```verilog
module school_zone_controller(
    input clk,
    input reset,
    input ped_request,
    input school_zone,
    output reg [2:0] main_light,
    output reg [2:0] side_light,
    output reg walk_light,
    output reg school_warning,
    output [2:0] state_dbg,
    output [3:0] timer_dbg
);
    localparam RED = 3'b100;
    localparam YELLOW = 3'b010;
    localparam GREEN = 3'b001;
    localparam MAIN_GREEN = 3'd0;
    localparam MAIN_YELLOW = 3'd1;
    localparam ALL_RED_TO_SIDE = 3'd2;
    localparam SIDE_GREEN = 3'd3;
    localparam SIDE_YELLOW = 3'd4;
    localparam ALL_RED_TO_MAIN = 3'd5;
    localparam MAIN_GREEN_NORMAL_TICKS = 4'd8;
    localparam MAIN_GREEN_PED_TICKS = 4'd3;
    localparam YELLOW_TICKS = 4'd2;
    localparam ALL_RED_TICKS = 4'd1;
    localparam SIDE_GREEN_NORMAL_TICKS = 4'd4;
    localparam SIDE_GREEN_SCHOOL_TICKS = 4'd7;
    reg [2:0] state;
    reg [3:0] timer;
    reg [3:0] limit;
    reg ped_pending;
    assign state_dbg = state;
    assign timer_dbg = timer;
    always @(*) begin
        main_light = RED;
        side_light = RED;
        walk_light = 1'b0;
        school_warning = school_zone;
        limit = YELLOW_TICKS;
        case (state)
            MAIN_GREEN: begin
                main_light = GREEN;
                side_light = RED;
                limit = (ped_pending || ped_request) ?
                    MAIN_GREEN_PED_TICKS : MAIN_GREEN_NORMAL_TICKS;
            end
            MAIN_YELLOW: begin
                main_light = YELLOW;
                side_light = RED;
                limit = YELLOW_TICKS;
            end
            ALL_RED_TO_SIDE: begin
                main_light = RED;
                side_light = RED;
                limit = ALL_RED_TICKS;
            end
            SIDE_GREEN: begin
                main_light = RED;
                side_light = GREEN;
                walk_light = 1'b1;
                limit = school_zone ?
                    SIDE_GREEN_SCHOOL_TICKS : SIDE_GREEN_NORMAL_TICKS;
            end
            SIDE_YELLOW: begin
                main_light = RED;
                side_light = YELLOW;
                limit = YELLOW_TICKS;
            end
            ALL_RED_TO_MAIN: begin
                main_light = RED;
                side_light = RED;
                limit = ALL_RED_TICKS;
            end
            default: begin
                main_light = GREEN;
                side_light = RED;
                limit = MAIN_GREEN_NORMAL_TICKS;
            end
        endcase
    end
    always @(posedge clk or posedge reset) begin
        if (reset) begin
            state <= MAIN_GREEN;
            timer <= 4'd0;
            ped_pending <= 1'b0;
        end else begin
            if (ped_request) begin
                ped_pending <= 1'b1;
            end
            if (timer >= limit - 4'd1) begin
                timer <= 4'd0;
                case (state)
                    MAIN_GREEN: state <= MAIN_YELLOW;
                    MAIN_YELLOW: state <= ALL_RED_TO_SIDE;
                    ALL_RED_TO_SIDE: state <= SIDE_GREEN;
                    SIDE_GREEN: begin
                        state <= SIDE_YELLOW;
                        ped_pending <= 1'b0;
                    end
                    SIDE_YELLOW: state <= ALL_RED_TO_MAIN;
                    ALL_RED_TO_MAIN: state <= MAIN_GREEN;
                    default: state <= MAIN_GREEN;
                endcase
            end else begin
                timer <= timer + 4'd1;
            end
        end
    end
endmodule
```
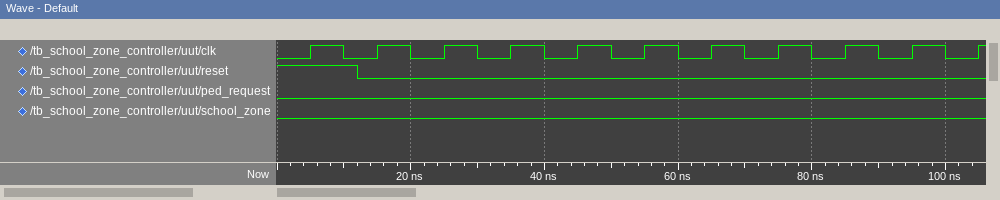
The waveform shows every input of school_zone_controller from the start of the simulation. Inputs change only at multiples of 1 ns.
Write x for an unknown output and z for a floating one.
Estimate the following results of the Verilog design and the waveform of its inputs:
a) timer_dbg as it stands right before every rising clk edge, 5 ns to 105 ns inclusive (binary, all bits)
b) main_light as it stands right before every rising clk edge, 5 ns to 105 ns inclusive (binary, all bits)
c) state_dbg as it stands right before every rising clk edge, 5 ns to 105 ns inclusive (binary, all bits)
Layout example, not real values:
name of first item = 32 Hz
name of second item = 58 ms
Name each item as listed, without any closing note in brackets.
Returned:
timer_dbg as it stands right before every rising clk edge, 5 ns to 105 ns inclusive = 0000, 0000, 0001, 0010, 0011, 0100, 0101, 0110, 0111, 0000, 0001
main_light as it stands right before every rising clk edge, 5 ns to 105 ns inclusive = 001, 001, 001, 001, 001, 001, 001, 001, 001, 010, 010
state_dbg as it stands right before every rising clk edge, 5 ns to 105 ns inclusive = 000, 000, 000, 000, 000, 000, 000, 000, 000, 001, 001
